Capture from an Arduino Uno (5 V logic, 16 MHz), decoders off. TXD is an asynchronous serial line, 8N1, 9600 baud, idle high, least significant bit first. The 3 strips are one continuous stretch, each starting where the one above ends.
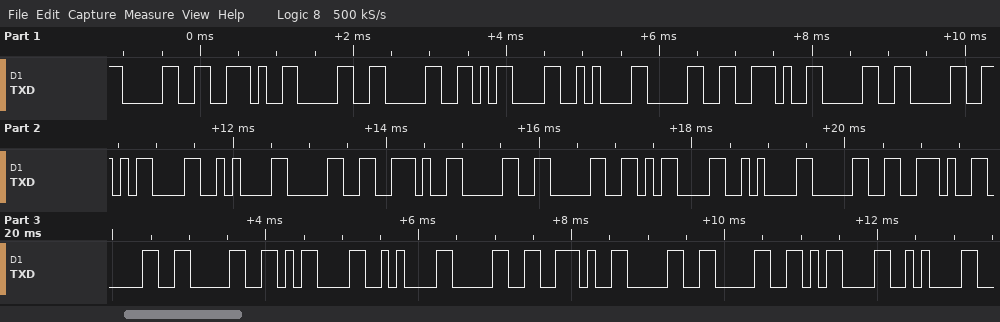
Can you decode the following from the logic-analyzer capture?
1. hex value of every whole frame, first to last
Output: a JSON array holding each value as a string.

["30 2E 30 30 0D 0A 30 2E 30 30 0D 0A 30 2E 30 30 0D 0A 30 2E 30 30 0D 0A 30 2E 30 30 0D 0A"]
